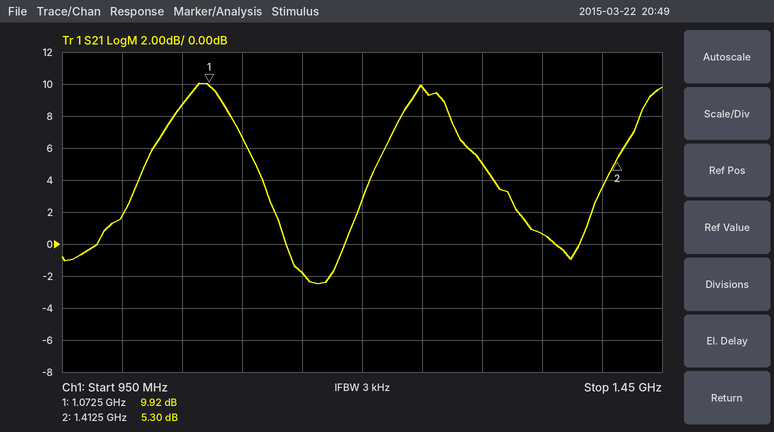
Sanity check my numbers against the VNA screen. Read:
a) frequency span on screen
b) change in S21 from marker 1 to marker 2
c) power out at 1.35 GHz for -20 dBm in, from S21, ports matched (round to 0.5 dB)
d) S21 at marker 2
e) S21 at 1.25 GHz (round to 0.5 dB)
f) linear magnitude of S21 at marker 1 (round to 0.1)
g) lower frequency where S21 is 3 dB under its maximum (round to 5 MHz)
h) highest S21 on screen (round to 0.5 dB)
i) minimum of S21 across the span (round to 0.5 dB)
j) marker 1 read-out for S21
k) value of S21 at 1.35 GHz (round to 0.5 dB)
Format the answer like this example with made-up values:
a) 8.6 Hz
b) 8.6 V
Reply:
a) 500 MHz
b) -4.62 dB
c) -19.5 dBm
d) 5.30 dB
e) 10.0 dB
f) 3.1
g) 1.035 GHz
h) 10.0 dB
i) -2.5 dB
j) 9.92 dB
k) 0.5 dB
